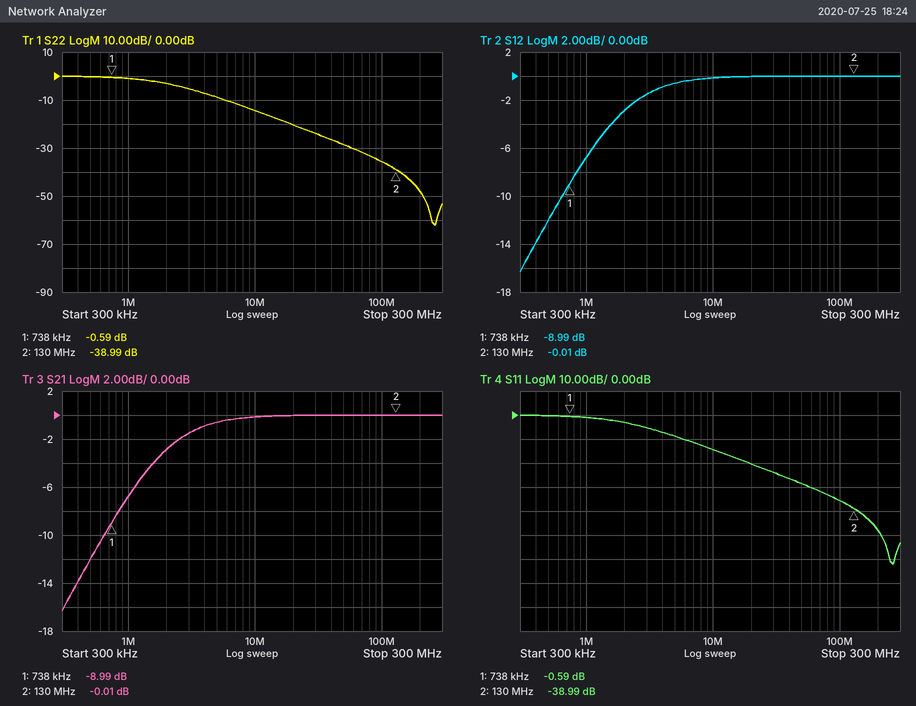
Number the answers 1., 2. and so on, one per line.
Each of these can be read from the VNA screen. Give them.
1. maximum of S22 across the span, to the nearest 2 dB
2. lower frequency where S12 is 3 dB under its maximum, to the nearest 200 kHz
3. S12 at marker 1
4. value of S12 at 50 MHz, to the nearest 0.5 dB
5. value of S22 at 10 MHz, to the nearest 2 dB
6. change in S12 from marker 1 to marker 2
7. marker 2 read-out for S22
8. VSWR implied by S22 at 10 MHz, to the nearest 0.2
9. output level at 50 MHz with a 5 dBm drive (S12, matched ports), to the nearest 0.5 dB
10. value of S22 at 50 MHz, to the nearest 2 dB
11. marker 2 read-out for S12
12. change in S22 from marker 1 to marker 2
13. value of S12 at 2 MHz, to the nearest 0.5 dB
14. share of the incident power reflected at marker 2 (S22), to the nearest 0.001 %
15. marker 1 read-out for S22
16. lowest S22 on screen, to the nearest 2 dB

1. 0 dB
2. 2.0 MHz
3. -8.99 dB
4. 0.0 dB
5. -14 dB
6. 8.98 dB
7. -38.99 dB
8. 1.4
9. 5.0 dBm
10. -28 dB
11. -0.01 dB
12. -38.40 dB
13. -3.0 dB
14. 0.013 %
15. -0.59 dB
16. -62 dB
